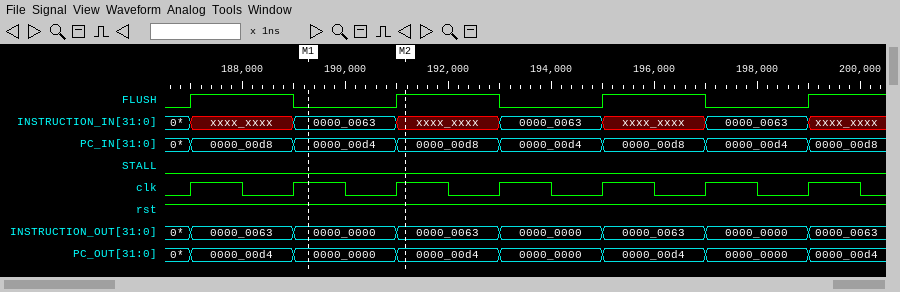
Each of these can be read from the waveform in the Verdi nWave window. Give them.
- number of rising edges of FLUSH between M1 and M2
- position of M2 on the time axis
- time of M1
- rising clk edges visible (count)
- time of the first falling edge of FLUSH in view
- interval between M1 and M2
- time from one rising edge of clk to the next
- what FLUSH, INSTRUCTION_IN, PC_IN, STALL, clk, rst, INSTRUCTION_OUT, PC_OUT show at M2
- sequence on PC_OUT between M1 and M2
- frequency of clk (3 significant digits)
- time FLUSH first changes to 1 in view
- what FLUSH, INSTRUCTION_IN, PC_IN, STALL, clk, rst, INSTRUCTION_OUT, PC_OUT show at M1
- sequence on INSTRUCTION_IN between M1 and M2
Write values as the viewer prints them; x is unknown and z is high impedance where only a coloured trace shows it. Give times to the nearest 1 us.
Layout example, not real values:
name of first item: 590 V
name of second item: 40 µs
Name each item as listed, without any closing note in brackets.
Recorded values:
number of rising edges of FLUSH between M1 and M2: 1
position of M2 on the time axis: 191 us
time of M1: 189 us
rising clk edges visible: 7
time of the first falling edge of FLUSH in view: 189 us
interval between M1 and M2: 2 us
time from one rising edge of clk to the next: 2 us
what FLUSH, INSTRUCTION_IN, PC_IN, STALL, clk, rst, INSTRUCTION_OUT, PC_OUT show at M2: FLUSH=1, INSTRUCTION_IN=xxxx_xxxx, PC_IN=0000_00d8, STALL=0, clk=1, rst=1, INSTRUCTION_OUT=0000_0063, PC_OUT=0000_00d4
sequence on PC_OUT between M1 and M2: 0000_0000, 0000_00d4
frequency of clk: 500 kHz
time FLUSH first changes to 1 in view: 187 us
what FLUSH, INSTRUCTION_IN, PC_IN, STALL, clk, rst, INSTRUCTION_OUT, PC_OUT show at M1: FLUSH=0, INSTRUCTION_IN=0000_0063, PC_IN=0000_00d4, STALL=0, clk=1, rst=1, INSTRUCTION_OUT=0000_0000, PC_OUT=0000_0000
sequence on INSTRUCTION_IN between M1 and M2: 0000_0063, xxxx_xxxx
